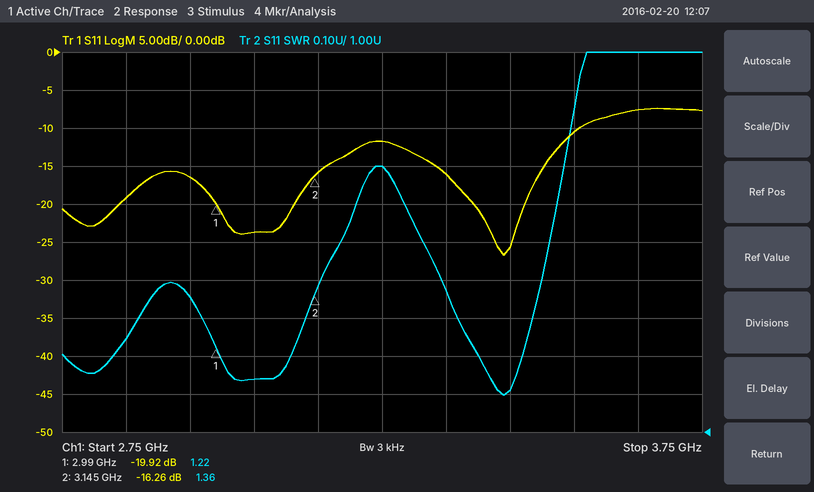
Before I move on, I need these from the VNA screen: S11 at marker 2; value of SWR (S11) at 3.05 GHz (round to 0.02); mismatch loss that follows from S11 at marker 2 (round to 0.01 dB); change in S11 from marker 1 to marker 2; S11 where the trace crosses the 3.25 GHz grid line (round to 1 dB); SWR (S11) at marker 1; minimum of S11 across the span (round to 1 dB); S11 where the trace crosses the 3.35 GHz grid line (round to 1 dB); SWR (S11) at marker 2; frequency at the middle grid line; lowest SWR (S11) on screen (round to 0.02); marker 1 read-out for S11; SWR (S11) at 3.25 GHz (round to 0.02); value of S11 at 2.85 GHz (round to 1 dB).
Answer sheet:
-16.26 dB
1.14
0.10 dB
3.66 dB
-12 dB
1.22
-27 dB
-16 dB
1.36
3.25 GHz
1.10
-19.92 dB
1.70
-19 dB
